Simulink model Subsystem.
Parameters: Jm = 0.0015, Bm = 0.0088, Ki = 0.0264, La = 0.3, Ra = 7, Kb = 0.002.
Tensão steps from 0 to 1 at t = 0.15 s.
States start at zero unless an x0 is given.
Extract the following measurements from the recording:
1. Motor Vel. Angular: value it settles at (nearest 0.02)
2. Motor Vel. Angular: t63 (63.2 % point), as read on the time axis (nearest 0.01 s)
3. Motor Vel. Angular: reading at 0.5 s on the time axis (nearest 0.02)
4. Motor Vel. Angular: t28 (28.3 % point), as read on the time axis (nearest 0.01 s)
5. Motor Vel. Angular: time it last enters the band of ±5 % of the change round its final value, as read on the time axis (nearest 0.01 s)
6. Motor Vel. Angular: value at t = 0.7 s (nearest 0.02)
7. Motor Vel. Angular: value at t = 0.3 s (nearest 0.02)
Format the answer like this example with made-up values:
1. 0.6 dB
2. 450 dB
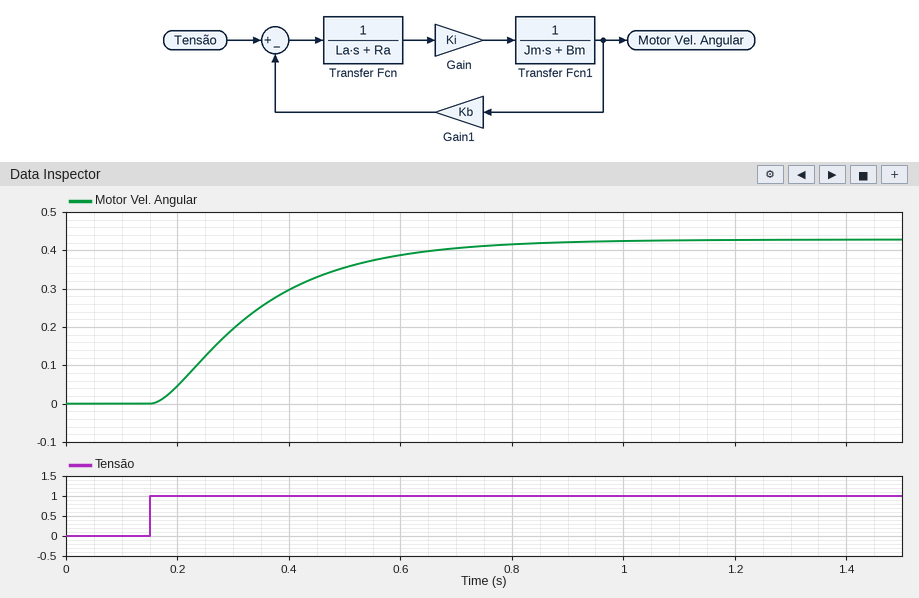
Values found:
1. 0.42
2. 0.37 s
3. 0.36
4. 0.25 s
5. 0.71 s
6. 0.40
7. 0.20
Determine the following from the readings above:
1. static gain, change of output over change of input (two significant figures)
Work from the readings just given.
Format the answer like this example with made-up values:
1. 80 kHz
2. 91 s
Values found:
1. 0.42
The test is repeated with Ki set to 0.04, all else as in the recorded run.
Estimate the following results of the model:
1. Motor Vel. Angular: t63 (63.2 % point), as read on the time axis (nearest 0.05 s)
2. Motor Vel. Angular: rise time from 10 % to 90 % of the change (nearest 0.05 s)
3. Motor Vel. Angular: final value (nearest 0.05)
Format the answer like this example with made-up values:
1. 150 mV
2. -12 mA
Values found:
1. 0.35 s
2. 0.40 s
3. 0.65
